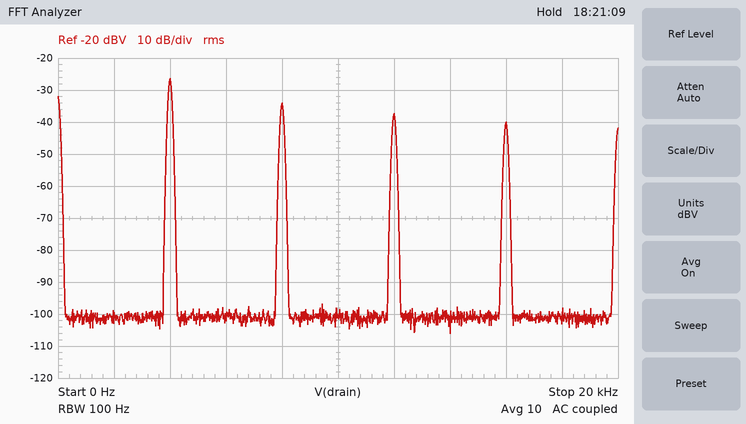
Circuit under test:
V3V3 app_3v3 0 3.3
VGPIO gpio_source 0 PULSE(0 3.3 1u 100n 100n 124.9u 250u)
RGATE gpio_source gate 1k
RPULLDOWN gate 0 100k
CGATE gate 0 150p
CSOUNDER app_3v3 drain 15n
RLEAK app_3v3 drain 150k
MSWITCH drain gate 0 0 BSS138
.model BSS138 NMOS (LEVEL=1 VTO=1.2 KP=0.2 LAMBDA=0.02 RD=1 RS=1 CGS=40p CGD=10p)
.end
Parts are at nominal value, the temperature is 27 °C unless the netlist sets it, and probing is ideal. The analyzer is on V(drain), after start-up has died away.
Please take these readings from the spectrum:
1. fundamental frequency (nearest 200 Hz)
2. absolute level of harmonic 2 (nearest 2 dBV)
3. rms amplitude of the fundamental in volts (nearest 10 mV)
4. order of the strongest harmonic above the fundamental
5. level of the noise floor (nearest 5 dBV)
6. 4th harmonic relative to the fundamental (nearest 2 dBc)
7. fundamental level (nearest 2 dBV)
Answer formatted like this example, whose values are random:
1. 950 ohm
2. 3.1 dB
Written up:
1. 4.0 kHz
2. -34 dBV
3. 50 mV
4. 2
5. -100 dBV
6. -14 dBc
7. -26 dBV
